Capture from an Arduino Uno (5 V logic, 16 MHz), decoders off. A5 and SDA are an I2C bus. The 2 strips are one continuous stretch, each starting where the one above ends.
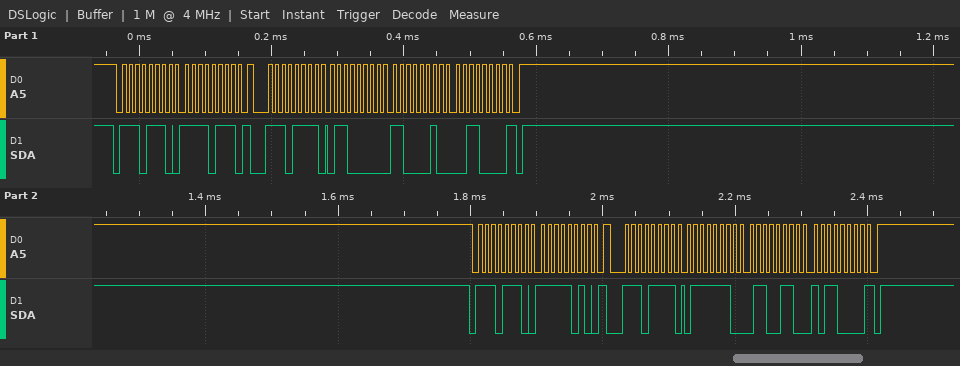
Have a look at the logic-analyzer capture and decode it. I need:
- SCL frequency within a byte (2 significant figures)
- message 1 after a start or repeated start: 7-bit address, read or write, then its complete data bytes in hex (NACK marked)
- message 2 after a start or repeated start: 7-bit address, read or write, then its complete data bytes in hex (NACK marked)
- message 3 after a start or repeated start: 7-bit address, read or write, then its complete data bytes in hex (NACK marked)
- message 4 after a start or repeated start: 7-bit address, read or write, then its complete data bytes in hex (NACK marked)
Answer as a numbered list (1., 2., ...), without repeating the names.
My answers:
1. 100 kHz
2. 0x77 write: F7
3. 0x77 read: 60 C2 30 NACK
4. 0x77 write: FA
5. 0x77 read: 7E 66 B0 NACK
